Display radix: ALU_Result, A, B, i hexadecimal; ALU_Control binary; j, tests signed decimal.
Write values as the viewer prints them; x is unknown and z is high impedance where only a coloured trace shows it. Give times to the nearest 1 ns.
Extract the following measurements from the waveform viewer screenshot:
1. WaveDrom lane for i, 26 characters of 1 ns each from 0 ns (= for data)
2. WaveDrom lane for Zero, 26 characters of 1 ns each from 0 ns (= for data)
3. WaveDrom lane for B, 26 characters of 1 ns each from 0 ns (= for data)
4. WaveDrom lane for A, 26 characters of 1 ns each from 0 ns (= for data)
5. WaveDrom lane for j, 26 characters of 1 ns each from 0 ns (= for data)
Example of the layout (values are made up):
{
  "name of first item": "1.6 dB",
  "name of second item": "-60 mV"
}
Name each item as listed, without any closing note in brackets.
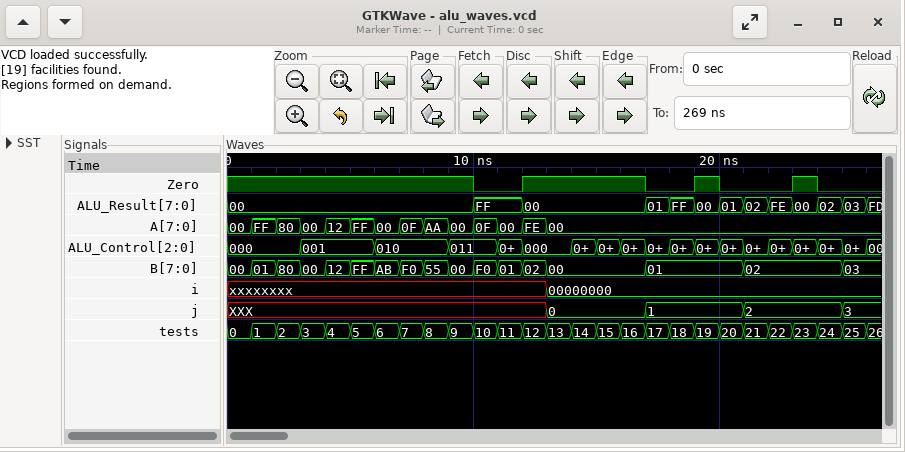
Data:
{
  "WaveDrom lane for i, 26 characters of 1 ns each from 0 ns": "{name: 'i', wave: 'x............=............', data: '00000000'}",
  "WaveDrom lane for Zero, 26 characters of 1 ns each from 0 ns": "{name: 'Zero', wave: '1.........0.1....0.10..10.'}",
  "WaveDrom lane for B, 26 characters of 1 ns each from 0 ns": "{name: 'B', wave: '==============...=...=...=', data: '00 01 80 00 12 FF AB F0 55 00 F0 01 02 00 01 02 03'}",
  "WaveDrom lane for A, 26 characters of 1 ns each from 0 ns": "{name: 'A', wave: '==============............', data: '00 FF 80 00 12 FF 00 0F AA 00 0F 00 FE 00'}",
  "WaveDrom lane for j, 26 characters of 1 ns each from 0 ns": "{name: 'j', wave: 'x............=...=...=...=', data: '0 1 2 3'}"
}
